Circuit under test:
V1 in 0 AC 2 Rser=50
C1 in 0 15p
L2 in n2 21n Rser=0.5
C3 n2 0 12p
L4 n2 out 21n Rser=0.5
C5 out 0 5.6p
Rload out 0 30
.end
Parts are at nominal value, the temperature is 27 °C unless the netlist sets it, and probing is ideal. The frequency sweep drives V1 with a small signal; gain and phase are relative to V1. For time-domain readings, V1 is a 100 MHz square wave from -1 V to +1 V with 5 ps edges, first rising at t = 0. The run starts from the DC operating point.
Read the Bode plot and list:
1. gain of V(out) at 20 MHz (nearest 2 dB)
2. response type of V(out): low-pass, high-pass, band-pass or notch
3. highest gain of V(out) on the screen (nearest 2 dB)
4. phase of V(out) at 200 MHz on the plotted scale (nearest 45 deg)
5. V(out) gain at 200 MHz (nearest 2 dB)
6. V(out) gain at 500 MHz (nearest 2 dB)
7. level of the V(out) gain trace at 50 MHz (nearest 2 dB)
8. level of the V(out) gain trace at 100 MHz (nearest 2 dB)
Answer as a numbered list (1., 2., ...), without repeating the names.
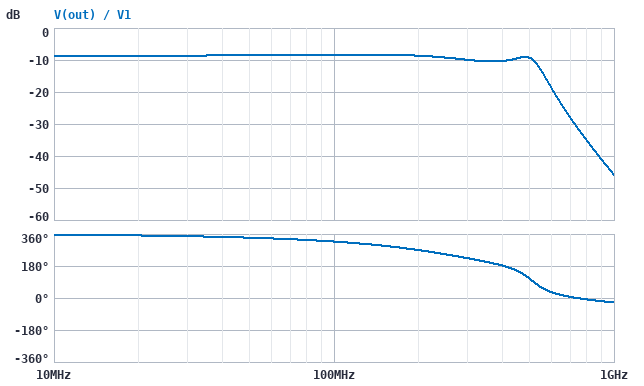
1. -8 dB
2. low-pass
3. -8 dB
4. 270 deg
5. -8 dB
6. -10 dB
7. -8 dB
8. -8 dB
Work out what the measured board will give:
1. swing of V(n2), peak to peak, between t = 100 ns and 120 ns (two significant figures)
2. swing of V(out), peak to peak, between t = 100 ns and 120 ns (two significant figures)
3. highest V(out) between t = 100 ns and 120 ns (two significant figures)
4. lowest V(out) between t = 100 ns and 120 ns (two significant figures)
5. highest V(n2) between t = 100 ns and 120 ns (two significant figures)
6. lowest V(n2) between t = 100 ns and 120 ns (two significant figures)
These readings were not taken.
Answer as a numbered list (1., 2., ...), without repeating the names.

1. 1.4 V
2. 940 mV
3. 470 mV
4. -470 mV
5. 690 mV
6. -690 mV
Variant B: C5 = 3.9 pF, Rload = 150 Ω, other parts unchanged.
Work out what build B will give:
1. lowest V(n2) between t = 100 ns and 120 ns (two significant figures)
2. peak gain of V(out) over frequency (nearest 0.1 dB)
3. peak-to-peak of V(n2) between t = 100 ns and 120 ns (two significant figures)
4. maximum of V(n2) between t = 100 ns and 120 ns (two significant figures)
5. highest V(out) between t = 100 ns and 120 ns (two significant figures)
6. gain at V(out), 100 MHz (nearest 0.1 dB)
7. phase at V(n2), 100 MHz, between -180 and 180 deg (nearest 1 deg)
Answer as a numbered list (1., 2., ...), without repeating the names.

1. -760 mV
2. -1.5 dB
3. 1.5 V
4. 760 mV
5. 820 mV
6. -3.5 dB
7. -40 deg
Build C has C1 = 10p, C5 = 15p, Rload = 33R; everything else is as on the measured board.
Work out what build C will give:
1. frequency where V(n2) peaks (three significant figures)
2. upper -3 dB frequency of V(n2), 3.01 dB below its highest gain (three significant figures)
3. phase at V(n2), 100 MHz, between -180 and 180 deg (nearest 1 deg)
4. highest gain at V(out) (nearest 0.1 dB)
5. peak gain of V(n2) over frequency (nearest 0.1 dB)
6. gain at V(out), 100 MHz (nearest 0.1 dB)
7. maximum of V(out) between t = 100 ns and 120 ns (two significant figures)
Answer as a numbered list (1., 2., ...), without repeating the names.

1. 522 MHz
2. 567 MHz
3. -20 deg
4. -8.0 dB
5. 1.2 dB
6. -8.1 dB
7. 500 mV
